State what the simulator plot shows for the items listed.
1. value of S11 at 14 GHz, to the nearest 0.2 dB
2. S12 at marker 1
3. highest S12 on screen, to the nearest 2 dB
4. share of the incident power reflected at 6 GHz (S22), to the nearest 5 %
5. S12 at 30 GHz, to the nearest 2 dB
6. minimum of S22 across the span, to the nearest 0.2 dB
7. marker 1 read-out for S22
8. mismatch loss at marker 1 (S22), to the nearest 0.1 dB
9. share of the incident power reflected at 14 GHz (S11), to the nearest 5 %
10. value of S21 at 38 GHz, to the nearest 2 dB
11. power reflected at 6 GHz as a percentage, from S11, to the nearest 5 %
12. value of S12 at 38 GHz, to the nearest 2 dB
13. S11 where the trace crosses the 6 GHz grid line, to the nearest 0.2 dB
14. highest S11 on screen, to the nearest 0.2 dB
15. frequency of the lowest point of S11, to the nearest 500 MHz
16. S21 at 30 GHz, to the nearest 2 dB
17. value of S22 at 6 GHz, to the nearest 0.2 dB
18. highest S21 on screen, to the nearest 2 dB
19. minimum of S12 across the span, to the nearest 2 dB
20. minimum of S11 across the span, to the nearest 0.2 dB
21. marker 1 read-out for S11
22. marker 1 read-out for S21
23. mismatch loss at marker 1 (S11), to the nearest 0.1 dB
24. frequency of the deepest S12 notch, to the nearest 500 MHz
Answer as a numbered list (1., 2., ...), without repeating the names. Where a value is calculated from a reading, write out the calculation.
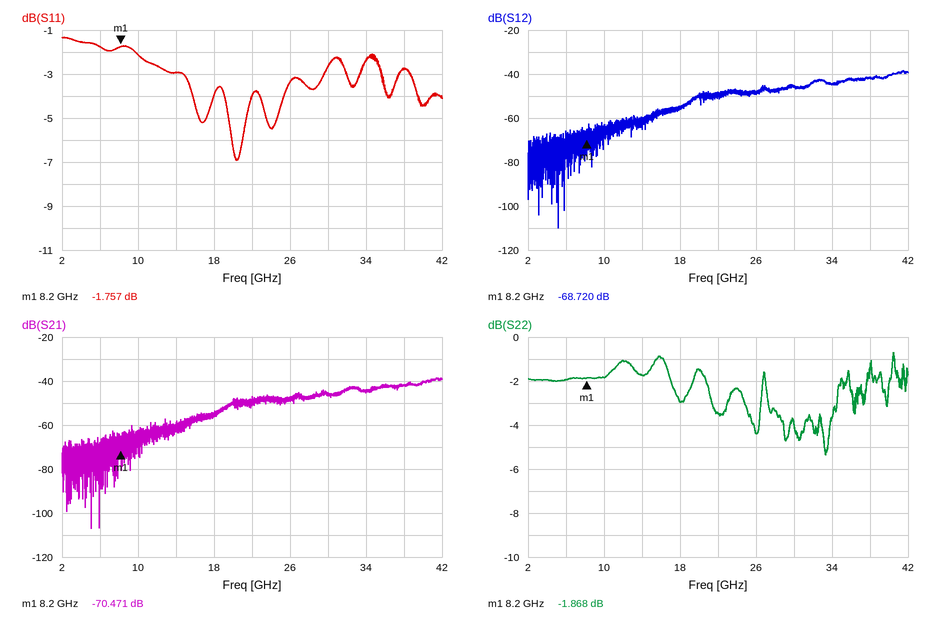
1. -3.0 dB
2. -68.720 dB
3. -38 dB
4. 10^(-2/10) ≈ 63.1 %, so 65 % to the nearest 5 %
5. -46 dB
6. -5.4 dB
7. -1.868 dB
8. −10 log10(1 − 10^(-1.868/10)) ≈ 4.6 dB
9. 10^(-3/10) ≈ 50 %
10. -42 dB
11. 10^(-1.8/10) ≈ 66.1 %, so 65 % to the nearest 5 %
12. -42 dB
13. -1.8 dB
14. -1.4 dB
15. 20.5 GHz
16. -46 dB
17. -2.0 dB
18. -38 dB
19. -110 dB
20. -7.0 dB
21. -1.757 dB
22. -70.471 dB
23. −10 log10(1 − 10^(-1.757/10)) ≈ 4.8 dB
24. 5.0 GHz
